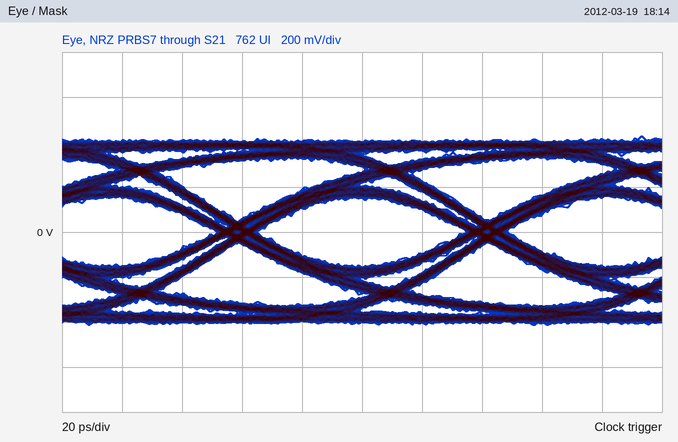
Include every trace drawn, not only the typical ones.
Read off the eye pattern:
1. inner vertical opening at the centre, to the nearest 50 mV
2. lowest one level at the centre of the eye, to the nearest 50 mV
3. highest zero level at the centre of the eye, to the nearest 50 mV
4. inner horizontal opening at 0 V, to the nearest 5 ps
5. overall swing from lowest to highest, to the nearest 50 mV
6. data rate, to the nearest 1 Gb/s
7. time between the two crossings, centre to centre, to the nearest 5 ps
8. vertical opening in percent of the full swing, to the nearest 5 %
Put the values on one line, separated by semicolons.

300 mV; 150 mV; -150 mV; 70 ps; 850 mV; 12 Gb/s; 85 ps; 35 %
